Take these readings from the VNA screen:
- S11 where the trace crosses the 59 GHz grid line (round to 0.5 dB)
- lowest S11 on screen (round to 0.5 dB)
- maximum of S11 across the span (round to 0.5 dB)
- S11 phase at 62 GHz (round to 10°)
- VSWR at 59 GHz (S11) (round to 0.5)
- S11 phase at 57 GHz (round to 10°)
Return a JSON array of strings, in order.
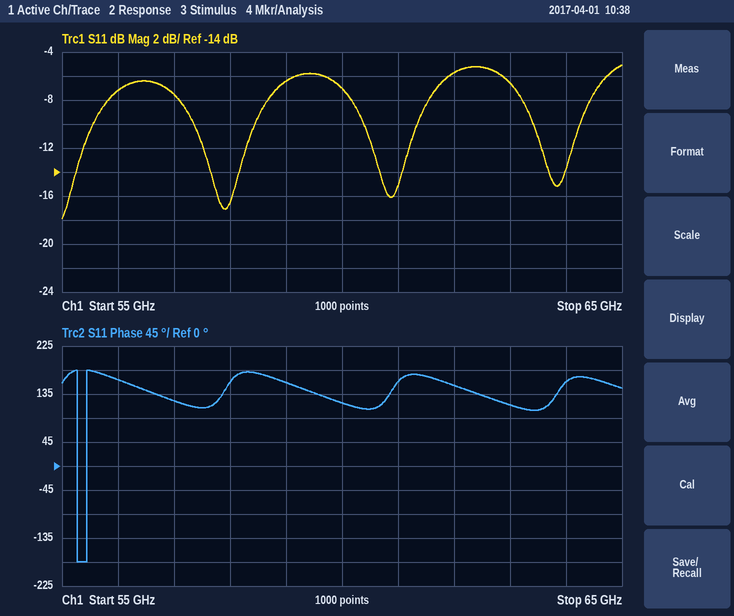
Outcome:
["-6.5 dB", "-18.0 dB", "-5.0 dB", "150°", "3.0", "120°"]
